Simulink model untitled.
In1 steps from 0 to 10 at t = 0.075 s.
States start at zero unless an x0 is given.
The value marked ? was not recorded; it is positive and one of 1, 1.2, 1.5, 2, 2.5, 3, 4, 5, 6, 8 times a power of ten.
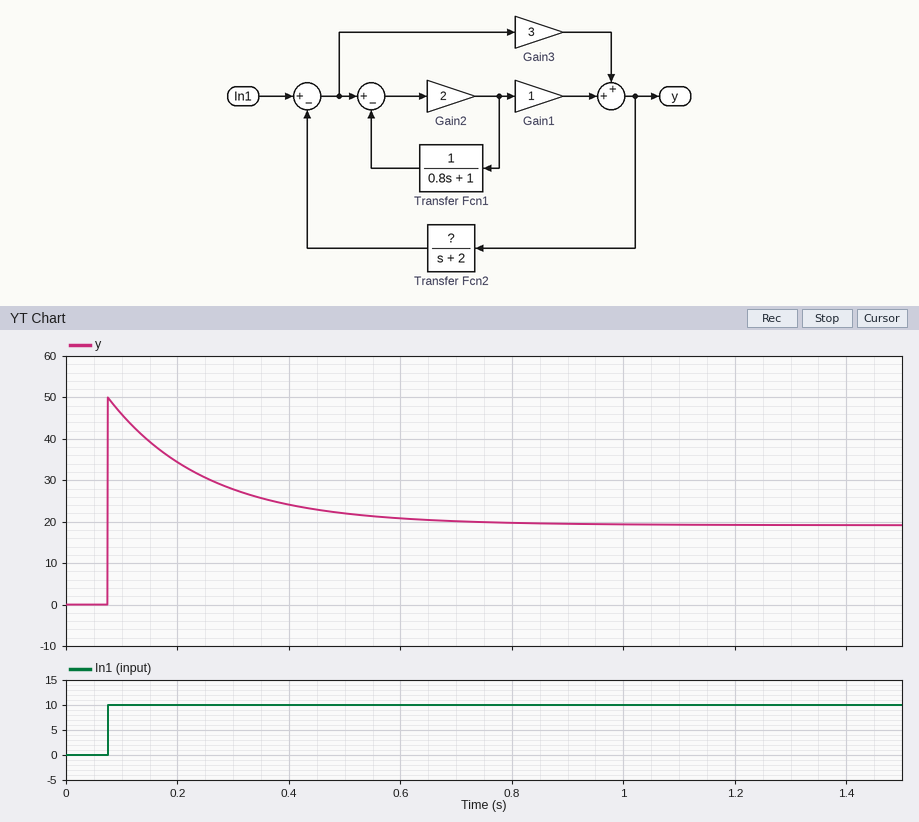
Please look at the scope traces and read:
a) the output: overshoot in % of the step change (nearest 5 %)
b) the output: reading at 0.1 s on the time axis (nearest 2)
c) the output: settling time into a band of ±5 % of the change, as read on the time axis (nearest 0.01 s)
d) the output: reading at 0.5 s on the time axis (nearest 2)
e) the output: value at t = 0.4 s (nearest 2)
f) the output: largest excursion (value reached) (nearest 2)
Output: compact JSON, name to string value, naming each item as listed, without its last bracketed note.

{"the output: overshoot in % of the step change": "160 %", "the output: reading at 0.1 s on the time axis": "46", "the output: settling time into a band of ±5 % of the change, as read on the time axis": "0.71 s", "the output: reading at 0.5 s on the time axis": "22", "the output: value at t = 0.4 s": "24", "the output: largest excursion (value reached)": "50"}
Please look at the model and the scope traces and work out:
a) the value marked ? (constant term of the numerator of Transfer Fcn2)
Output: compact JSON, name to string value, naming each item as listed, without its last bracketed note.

{"the value marked ?": "0.5"}
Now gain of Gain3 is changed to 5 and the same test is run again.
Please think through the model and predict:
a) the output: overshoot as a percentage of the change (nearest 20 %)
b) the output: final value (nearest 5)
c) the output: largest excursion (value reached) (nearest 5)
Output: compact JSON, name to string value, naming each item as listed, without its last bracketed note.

{"the output: overshoot as a percentage of the change": "200 %", "the output: final value": "25", "the output: largest excursion (value reached)": "70"}
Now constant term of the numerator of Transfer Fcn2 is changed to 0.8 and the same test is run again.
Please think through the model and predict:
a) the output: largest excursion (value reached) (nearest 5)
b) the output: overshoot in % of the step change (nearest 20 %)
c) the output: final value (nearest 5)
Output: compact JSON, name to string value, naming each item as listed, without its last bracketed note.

{"the output: largest excursion (value reached)": "50", "the output: overshoot in % of the step change": "240 %", "the output: final value": "15"}
